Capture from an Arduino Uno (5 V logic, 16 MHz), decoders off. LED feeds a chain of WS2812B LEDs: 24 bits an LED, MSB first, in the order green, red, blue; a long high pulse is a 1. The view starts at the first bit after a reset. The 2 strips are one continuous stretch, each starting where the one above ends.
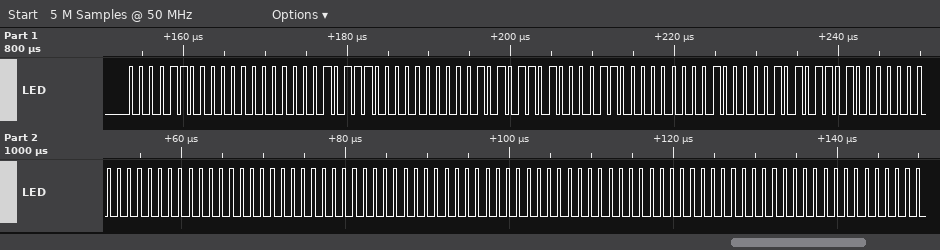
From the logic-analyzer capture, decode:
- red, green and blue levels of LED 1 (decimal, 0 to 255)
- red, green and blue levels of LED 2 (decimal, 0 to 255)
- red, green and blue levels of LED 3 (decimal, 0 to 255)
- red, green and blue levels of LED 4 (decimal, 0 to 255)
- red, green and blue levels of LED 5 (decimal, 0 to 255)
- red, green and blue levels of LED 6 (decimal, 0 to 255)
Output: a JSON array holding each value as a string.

["0, 12, 23", "43, 0, 67", "65, 0, 90", "0, 0, 0", "0, 0, 0", "0, 0, 0"]
